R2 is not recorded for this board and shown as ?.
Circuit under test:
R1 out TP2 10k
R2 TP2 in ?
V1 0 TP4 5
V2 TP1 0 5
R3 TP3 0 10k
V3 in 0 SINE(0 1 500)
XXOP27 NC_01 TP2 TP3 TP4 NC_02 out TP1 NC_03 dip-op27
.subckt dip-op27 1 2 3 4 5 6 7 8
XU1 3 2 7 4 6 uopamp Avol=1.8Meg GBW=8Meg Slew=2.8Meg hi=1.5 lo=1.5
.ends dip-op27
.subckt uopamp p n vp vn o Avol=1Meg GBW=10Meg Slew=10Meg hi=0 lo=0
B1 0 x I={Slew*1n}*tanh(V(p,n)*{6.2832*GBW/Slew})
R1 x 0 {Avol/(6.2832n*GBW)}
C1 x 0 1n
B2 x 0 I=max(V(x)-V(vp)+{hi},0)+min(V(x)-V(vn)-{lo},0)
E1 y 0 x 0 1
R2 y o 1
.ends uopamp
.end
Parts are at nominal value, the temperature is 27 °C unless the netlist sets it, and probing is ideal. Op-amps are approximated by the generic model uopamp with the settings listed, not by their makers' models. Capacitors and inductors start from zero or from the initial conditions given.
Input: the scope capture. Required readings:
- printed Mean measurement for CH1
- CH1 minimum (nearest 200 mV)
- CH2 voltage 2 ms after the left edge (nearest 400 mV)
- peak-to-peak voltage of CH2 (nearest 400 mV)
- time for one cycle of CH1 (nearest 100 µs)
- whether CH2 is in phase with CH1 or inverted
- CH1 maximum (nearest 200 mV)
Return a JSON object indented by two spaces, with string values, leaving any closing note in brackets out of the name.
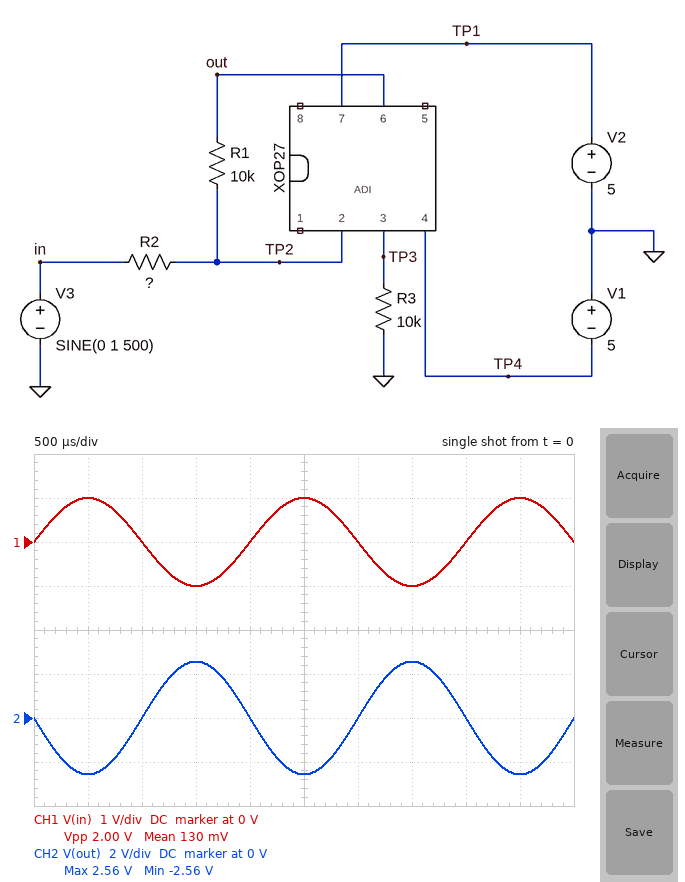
{
  "printed Mean measurement for CH1": "130 mV",
  "CH1 minimum": "-1.0 V",
  "CH2 voltage 2 ms after the left edge": "0 V",
  "peak-to-peak voltage of CH2": "5.2 V",
  "time for one cycle of CH1": "2.0 ms",
  "whether CH2 is in phase with CH1 or inverted": "inverted",
  "CH1 maximum": "1.0 V"
}
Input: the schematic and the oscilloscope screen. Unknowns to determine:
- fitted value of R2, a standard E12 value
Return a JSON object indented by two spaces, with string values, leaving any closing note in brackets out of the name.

{
  "fitted value of R2, a standard E12 value": "3.9 kΩ"
}
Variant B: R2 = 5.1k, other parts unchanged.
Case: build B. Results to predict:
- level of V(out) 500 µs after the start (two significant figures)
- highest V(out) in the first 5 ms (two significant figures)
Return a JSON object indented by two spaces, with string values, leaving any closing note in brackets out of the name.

{
  "level of V(out) 500 µs after the start": "-2.0 V",
  "highest V(out) in the first 5 ms": "2.0 V"
}
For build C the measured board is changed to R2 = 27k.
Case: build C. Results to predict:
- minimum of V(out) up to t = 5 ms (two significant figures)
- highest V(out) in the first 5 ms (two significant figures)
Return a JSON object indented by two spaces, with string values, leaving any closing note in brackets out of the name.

{
  "minimum of V(out) up to t = 5 ms": "-370 mV",
  "highest V(out) in the first 5 ms": "370 mV"
}
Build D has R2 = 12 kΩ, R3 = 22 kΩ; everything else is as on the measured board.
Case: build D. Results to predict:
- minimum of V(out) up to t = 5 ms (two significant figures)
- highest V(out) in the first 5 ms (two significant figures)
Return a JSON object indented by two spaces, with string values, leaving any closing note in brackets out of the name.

{
  "minimum of V(out) up to t = 5 ms": "-830 mV",
  "highest V(out) in the first 5 ms": "830 mV"
}
